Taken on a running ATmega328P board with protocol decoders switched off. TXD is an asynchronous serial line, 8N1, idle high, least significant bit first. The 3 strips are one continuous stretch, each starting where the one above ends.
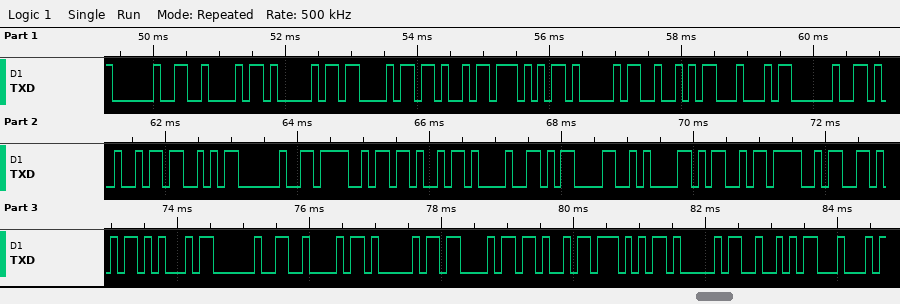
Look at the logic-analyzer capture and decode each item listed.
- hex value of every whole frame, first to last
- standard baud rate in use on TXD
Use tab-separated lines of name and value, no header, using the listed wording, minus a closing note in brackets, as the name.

hex value of every whole frame, first to last	0x20 0x42 0x41 0x43 0x4B 0x57 0x41 0x52 0x44 0x20 0x49 0x53 0x20 0x4F 0x4B 0x21 0x0D 0x0A 0x4D 0x4F 0x56 0x45 0x20 0x42 0x41 0x43 0x4B 0x57 0x41 0x52 0x44
standard baud rate in use on TXD	9600 baud
